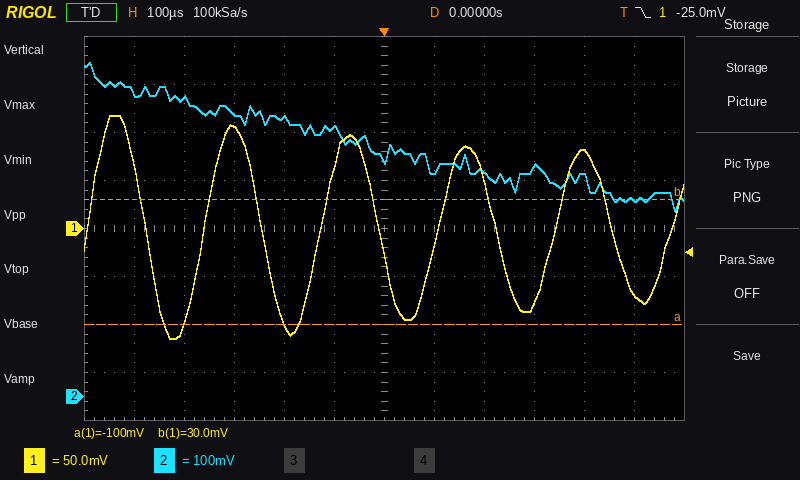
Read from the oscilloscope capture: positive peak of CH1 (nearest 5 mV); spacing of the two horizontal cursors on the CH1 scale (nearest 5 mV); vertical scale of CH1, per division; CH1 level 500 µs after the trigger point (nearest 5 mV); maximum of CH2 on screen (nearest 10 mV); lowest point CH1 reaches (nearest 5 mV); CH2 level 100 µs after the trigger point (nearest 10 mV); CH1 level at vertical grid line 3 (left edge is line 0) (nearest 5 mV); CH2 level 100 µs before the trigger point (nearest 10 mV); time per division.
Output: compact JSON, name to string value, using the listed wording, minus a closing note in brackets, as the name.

{"positive peak of CH1": "120 mV", "spacing of the two horizontal cursors on the CH1 scale": "130 mV", "vertical scale of CH1, per division": "50 mV", "CH1 level 500 µs after the trigger point": "-70 mV", "maximum of CH2 on screen": "700 mV", "lowest point CH1 reaches": "-115 mV", "CH2 level 100 µs after the trigger point": "470 mV", "CH1 level at vertical grid line 3 (left edge is line 0)": "105 mV", "CH2 level 100 µs before the trigger point": "560 mV", "time per division": "100 µs"}
